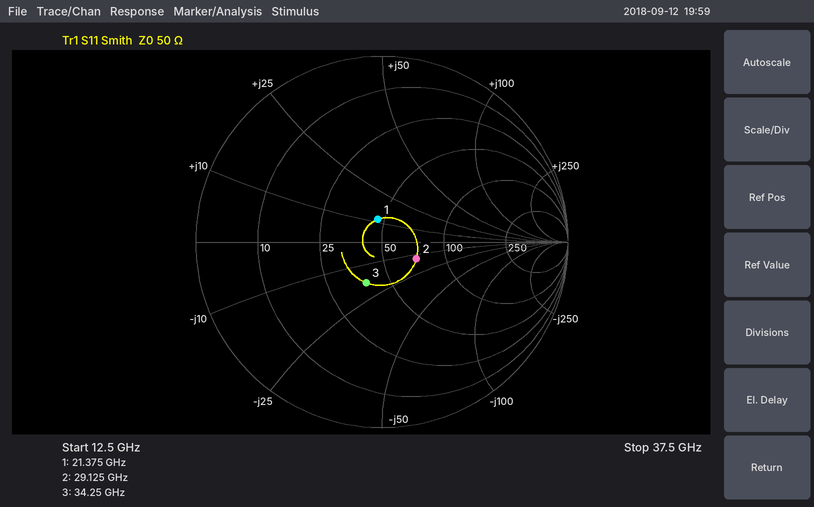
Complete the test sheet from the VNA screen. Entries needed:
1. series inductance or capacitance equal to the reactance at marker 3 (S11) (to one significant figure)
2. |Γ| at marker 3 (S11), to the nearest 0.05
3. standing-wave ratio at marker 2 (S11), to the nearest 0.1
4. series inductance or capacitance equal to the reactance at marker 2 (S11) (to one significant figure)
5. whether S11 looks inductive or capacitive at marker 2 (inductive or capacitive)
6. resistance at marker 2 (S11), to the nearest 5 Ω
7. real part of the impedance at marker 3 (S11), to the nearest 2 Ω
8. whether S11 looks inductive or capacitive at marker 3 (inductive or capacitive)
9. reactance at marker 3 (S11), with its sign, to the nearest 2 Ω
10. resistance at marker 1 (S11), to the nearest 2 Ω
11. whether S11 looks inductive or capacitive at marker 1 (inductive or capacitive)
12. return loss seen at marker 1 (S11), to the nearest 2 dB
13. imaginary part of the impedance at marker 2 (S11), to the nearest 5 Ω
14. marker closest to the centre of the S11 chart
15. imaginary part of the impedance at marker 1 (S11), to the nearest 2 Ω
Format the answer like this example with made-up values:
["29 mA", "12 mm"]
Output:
["300 fF", "0.25", "1.5", "400 fF", "capacitive", "70 Ω", "38 Ω", "capacitive", "-18 Ω", "46 Ω", "inductive", "18 dB", "-15 Ω", "marker 1", "+12 Ω"]
